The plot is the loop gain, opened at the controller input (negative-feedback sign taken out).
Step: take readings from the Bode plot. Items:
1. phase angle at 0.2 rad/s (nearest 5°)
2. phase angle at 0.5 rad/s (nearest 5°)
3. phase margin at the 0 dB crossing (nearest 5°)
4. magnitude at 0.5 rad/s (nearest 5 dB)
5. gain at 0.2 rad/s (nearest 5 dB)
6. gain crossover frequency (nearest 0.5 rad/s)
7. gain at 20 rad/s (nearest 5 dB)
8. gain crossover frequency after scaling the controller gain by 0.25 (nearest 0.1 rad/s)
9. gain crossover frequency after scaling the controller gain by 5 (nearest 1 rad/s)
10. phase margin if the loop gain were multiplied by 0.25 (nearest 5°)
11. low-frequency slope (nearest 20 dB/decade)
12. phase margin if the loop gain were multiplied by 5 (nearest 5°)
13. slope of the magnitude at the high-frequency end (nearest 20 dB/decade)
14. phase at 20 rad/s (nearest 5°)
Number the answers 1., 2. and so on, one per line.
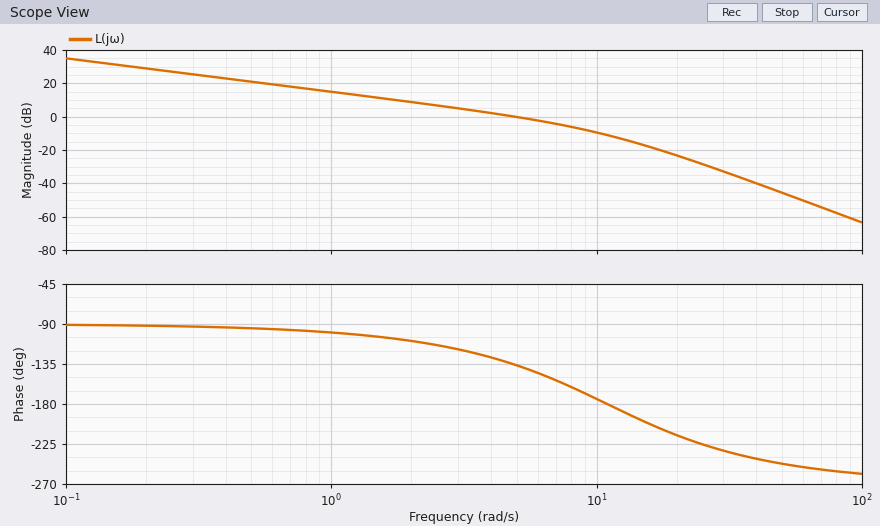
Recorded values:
1. -90°
2. -95°
3. 45°
4. 20 dB
5. 30 dB
6. 5.0 rad/s
7. -25 dB
8. 1.4 rad/s
9. 13 rad/s
10. 75°
11. -20 dB/decade
12. -10°
13. -60 dB/decade
14. -215°
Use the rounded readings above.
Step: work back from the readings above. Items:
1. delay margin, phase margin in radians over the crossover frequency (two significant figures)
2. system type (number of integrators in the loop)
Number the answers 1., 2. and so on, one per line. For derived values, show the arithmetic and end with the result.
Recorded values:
1. 45 × π / 180 / 5 = 0.16 s
2. 1
